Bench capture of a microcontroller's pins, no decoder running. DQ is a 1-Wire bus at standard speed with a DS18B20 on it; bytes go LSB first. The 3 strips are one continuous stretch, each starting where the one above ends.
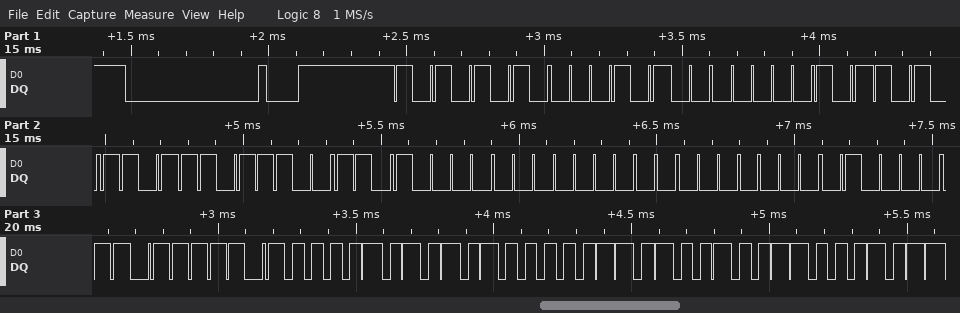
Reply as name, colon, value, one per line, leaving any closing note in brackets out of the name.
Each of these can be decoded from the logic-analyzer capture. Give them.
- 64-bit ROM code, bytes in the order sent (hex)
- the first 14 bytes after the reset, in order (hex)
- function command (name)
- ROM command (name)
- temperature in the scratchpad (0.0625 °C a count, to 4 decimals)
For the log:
64-bit ROM code, bytes in the order sent: 28 A0 B5 3B 0B 00 00 C2
the first 14 bytes after the reset, in order: 55 28 A0 B5 3B 0B 00 00 C2 BE 50 05 4B 46
function command: Read Scratchpad
ROM command: Match ROM
temperature in the scratchpad: 85.0000 °C
